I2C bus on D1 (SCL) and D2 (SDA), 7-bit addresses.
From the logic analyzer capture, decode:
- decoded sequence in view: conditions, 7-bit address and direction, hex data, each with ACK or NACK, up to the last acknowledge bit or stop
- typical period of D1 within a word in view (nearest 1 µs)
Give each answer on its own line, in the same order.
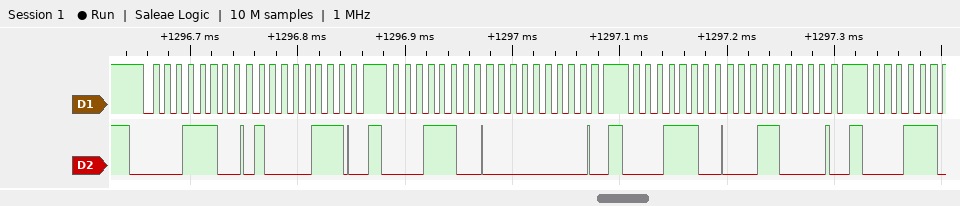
start, address 0E write ACK, 87 ACK, stop, start, address 0E write ACK, 00 ACK, stop, start, address 0E write ACK, 30 ACK, stop
11 µs
